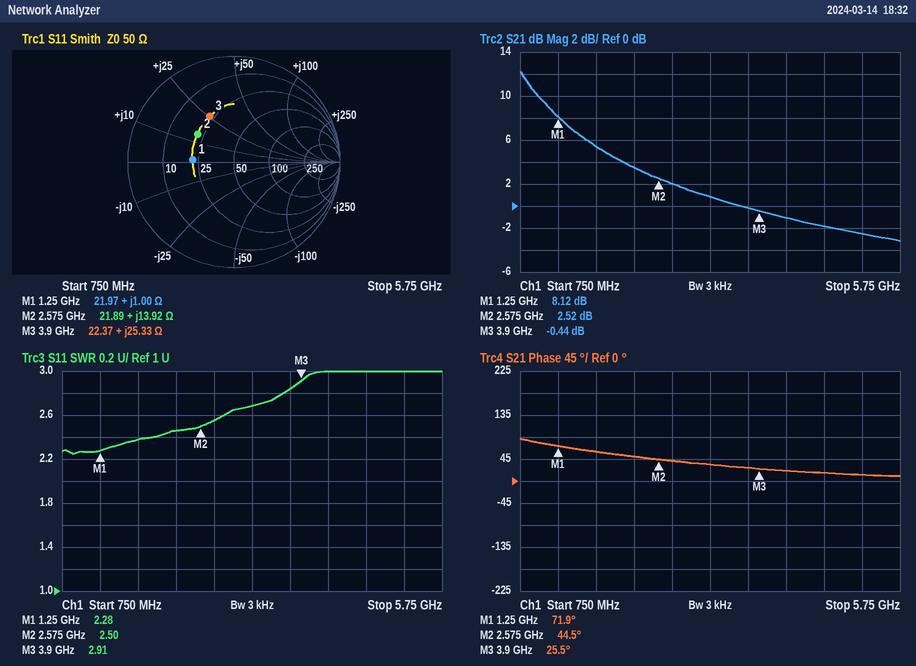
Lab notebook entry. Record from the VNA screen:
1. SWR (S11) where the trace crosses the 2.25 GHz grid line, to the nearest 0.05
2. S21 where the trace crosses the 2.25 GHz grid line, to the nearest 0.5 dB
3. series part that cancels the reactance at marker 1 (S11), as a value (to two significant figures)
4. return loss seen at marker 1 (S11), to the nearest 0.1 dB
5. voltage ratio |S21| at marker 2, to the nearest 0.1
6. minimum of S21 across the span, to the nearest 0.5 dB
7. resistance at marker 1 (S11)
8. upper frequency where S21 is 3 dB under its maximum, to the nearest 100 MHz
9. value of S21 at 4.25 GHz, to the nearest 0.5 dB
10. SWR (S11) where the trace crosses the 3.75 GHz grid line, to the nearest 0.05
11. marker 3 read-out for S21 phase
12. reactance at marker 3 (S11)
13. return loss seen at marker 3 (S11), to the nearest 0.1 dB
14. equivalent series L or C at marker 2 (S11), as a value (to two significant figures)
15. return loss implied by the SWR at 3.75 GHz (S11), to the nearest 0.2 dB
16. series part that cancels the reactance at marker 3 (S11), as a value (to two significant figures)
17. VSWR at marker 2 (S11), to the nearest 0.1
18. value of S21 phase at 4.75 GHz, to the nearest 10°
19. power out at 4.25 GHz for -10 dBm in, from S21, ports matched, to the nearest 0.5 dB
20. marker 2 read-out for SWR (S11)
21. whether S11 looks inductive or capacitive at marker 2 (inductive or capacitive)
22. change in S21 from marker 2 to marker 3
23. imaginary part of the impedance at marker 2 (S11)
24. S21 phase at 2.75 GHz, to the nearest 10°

2.45
3.5 dB
130 pF
8.2 dB
1.3
-3.0 dB
21.97 Ω
1.1 GHz
-1.0 dB
2.85
25.5°
+25.33 Ω
6.2 dB
860 pH
6.4 dB
1.6 pF
2.5
20°
-11.0 dBm
2.50
inductive
-2.96 dB
+13.92 Ω
40°
